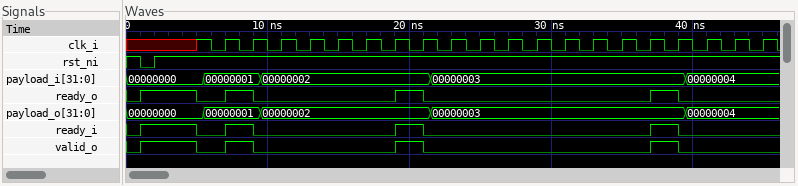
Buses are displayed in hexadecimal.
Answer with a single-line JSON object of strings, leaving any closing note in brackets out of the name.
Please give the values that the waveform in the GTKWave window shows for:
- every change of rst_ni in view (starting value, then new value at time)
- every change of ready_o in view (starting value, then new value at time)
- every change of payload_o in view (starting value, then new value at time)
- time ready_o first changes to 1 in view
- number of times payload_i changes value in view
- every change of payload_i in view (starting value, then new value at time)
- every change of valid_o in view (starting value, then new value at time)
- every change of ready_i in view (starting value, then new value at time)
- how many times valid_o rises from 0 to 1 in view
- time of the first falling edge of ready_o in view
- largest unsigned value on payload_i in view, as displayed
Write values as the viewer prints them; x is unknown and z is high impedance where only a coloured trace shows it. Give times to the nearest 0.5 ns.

{"every change of rst_ni in view": "1, 0 at 1 ns, 1 at 2 ns", "every change of ready_o in view": "0, 1 at 1 ns, 0 at 5 ns, 1 at 7 ns, 0 at 9 ns, 1 at 19 ns, 0 at 21 ns, 1 at 37 ns, 0 at 39 ns", "every change of payload_o in view": "00000000, 00000001 at 5.5 ns, 00000002 at 9.5 ns, 00000003 at 21.5 ns, 00000004 at 39.5 ns", "time ready_o first changes to 1 in view": "1 ns", "number of times payload_i changes value in view": "4", "every change of payload_i in view": "00000000, 00000001 at 5.5 ns, 00000002 at 9.5 ns, 00000003 at 21.5 ns, 00000004 at 39.5 ns", "every change of valid_o in view": "0, 1 at 1 ns, 0 at 5 ns, 1 at 7 ns, 0 at 9 ns, 1 at 19 ns, 0 at 21 ns, 1 at 37 ns, 0 at 39 ns", "every change of ready_i in view": "0, 1 at 1 ns, 0 at 5 ns, 1 at 7 ns, 0 at 9 ns, 1 at 19 ns, 0 at 21 ns, 1 at 37 ns, 0 at 39 ns", "how many times valid_o rises from 0 to 1 in view": "4", "time of the first falling edge of ready_o in view": "5 ns", "largest unsigned value on payload_i in view, as displayed": "00000004"}
